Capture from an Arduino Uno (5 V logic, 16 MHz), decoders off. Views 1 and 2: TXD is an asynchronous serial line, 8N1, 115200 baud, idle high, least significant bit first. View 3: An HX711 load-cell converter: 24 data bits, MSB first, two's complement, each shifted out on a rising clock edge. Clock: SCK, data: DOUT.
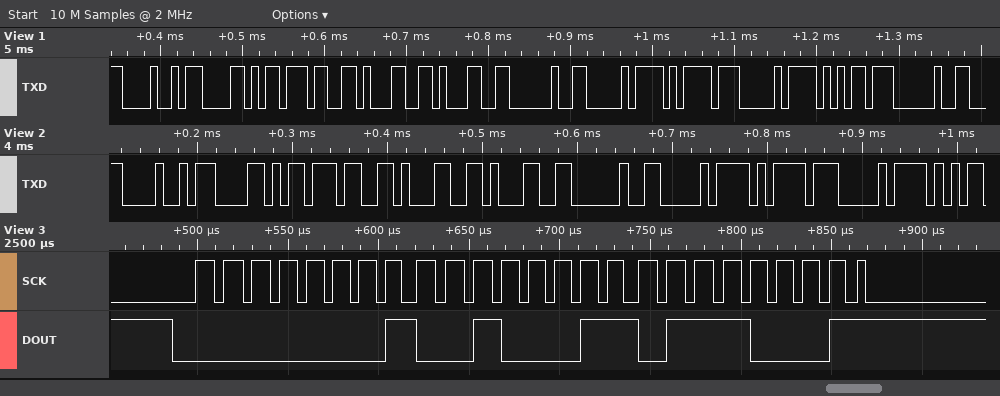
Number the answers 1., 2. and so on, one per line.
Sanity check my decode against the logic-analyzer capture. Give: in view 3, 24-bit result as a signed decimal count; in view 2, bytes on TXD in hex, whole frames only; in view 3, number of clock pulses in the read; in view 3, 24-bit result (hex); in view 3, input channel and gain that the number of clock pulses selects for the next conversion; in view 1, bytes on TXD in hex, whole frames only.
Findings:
1. 74609
2. 48 58 37 31 31 20 D0 BD D0
3. 25
4. 0x012371
5. channel A, gain 128
6. 48 58 37 31 31 20 D0 BD D0 B5 20
